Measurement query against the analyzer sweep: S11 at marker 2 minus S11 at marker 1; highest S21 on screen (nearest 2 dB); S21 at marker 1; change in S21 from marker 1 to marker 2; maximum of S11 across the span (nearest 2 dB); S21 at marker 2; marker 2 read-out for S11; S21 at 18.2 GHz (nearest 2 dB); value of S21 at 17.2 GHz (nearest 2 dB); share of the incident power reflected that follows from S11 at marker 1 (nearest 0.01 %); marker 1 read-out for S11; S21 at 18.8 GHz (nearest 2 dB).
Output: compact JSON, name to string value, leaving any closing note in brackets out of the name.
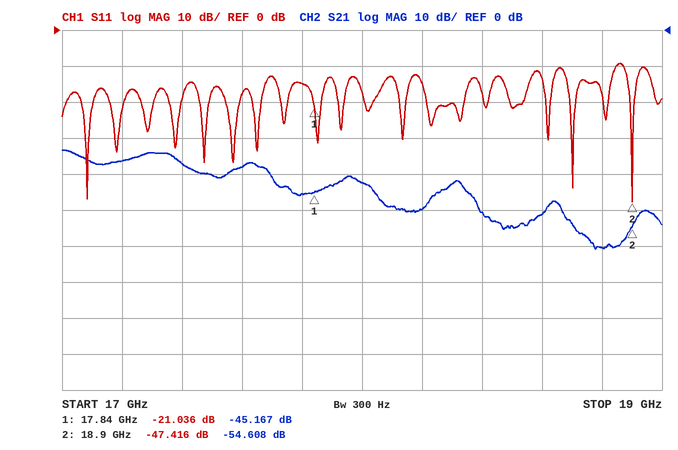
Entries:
{"S11 at marker 2 minus S11 at marker 1": "-26.380 dB", "highest S21 on screen": "-34 dB", "S21 at marker 1": "-45.167 dB", "change in S21 from marker 1 to marker 2": "-9.441 dB", "maximum of S11 across the span": "-10 dB", "S21 at marker 2": "-54.608 dB", "marker 2 read-out for S11": "-47.416 dB", "S21 at 18.2 GHz": "-50 dB", "value of S21 at 17.2 GHz": "-36 dB", "share of the incident power reflected that follows from S11 at marker 1": "0.79 %", "marker 1 read-out for S11": "-21.036 dB", "S21 at 18.8 GHz": "-60 dB"}
